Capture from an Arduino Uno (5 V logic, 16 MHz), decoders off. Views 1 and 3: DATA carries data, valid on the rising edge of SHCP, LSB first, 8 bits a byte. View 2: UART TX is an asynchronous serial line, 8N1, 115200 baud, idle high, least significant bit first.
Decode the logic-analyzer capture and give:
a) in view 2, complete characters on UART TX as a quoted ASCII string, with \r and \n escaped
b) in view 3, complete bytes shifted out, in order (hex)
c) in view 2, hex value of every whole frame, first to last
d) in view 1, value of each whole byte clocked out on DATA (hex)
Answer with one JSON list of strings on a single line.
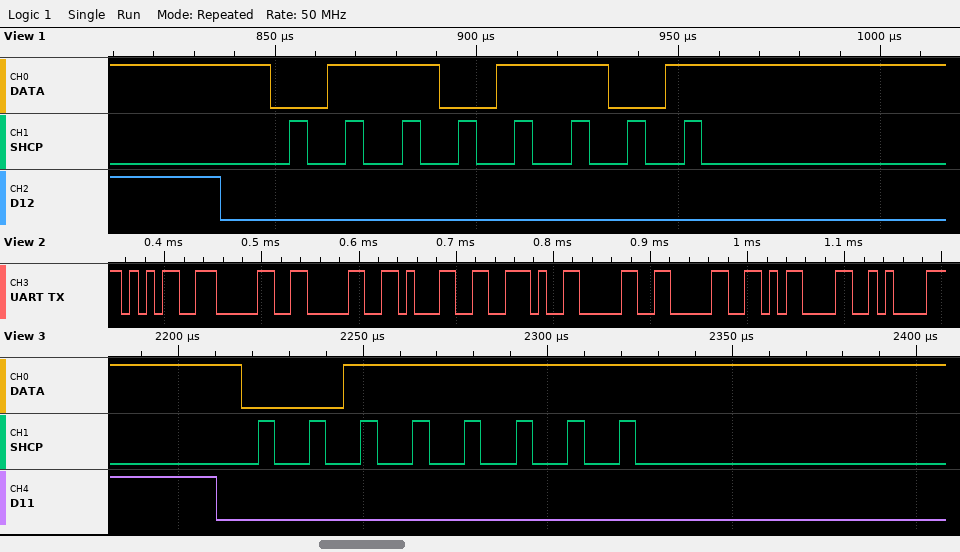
["\"5001.00\\r\\n\"", "FC", "0x35 0x30 0x30 0x31 0x2E 0x30 0x30 0x0D 0x0A", "B6"]
